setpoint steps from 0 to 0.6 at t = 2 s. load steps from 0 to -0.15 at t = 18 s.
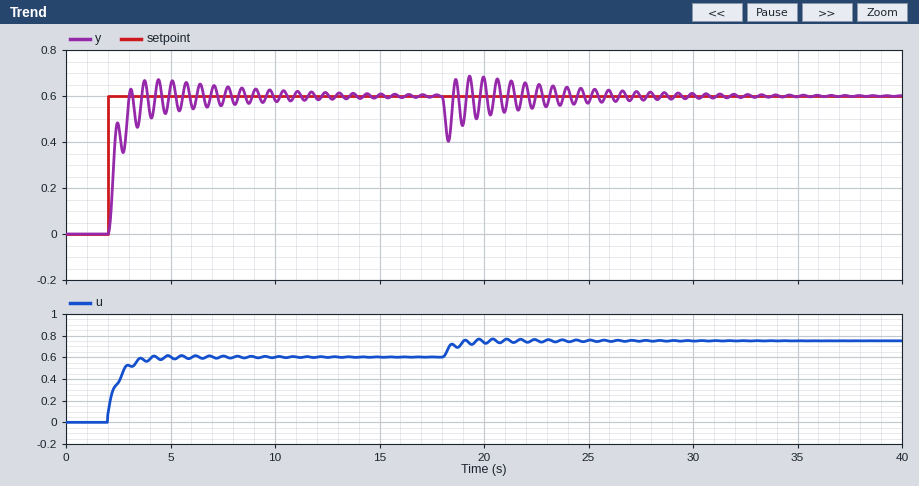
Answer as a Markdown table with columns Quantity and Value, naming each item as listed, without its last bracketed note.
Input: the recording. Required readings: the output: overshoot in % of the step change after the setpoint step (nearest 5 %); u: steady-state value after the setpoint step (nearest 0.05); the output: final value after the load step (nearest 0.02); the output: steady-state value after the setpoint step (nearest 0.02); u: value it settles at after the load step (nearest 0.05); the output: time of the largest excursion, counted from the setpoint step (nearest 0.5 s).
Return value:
| Quantity | Value |
|---|---|
| the output: overshoot in % of the step change after the setpoint step | 10 % |
| u: steady-state value after the setpoint step | 0.60 |
| the output: final value after the load step | 0.60 |
| the output: steady-state value after the setpoint step | 0.60 |
| u: value it settles at after the load step | 0.75 |
| the output: time of the largest excursion, counted from the setpoint step | 2.5 s |
